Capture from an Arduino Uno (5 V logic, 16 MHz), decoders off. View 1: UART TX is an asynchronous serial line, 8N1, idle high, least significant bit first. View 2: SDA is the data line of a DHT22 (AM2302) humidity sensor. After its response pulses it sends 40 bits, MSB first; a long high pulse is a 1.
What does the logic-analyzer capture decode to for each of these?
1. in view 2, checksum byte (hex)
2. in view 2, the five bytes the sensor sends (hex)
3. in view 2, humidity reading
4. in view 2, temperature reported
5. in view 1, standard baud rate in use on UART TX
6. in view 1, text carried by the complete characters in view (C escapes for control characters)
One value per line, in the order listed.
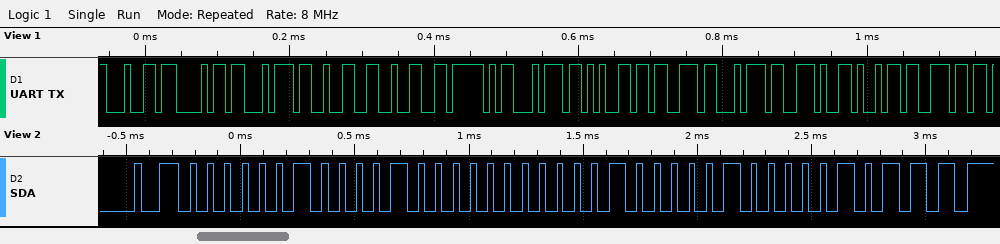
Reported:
0x17
02 10 01 04 17
52.8 %
26.0 °C
115200 baud
"dht22_test.in"
